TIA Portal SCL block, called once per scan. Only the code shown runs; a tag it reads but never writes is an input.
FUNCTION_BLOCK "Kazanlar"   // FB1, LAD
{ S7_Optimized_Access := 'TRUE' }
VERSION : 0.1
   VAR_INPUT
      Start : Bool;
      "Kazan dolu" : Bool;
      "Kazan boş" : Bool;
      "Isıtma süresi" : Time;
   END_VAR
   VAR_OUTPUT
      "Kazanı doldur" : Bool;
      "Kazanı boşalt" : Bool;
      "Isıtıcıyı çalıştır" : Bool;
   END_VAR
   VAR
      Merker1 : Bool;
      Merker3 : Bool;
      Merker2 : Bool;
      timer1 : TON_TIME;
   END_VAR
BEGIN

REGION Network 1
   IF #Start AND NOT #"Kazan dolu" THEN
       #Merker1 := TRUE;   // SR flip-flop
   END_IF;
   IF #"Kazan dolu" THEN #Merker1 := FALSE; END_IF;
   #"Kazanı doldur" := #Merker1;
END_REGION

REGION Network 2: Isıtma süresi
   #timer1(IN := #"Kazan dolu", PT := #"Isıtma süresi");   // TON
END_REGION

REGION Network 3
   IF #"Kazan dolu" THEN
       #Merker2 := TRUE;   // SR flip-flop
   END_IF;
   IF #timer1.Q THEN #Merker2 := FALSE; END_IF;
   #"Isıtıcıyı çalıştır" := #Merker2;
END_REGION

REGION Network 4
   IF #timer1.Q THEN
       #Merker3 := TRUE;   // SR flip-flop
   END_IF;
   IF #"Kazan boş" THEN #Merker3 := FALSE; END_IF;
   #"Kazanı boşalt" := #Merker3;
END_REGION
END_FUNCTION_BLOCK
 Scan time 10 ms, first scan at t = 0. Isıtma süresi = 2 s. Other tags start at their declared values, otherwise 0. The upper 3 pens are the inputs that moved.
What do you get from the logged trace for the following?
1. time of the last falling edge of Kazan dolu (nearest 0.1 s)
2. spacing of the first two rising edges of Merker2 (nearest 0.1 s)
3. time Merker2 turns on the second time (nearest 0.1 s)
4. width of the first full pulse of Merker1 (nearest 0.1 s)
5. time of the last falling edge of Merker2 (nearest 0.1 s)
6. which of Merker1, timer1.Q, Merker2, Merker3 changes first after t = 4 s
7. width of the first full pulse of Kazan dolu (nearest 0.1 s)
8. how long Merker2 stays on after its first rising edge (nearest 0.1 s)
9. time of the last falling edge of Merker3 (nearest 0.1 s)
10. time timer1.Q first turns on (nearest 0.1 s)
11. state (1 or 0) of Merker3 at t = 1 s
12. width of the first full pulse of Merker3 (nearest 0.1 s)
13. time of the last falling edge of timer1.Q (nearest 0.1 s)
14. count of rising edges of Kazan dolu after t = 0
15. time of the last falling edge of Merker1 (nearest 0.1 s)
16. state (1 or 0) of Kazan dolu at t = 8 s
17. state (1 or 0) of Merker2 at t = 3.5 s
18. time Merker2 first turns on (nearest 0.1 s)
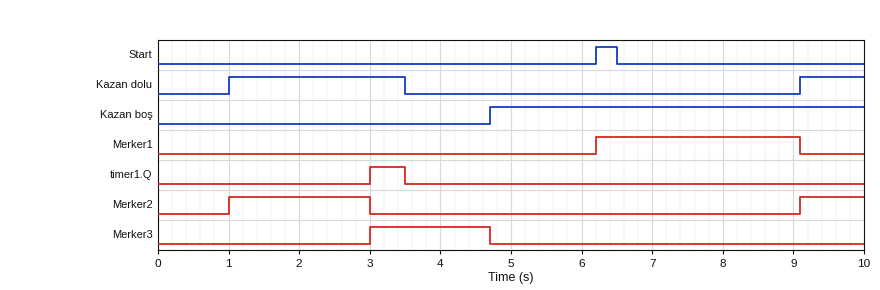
3.5 s
8.1 s
9.1 s
2.9 s
3.0 s
Merker3
2.5 s
2.0 s
4.7 s
3.0 s
0
1.7 s
3.5 s
2
9.1 s
0
0
1.0 s
